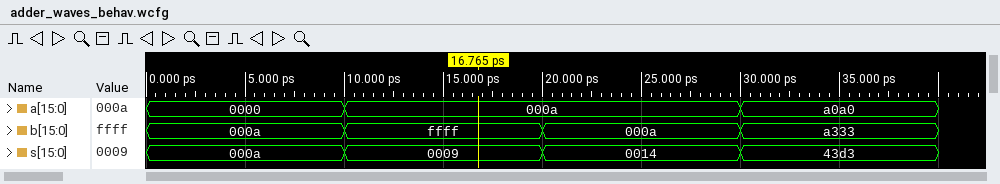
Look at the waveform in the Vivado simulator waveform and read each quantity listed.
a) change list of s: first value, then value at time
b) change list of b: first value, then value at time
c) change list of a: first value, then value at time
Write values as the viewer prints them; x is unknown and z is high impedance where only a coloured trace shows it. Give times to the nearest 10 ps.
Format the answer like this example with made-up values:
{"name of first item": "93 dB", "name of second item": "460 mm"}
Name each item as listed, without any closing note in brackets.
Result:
{"change list of s: first value, then value at time": "000a, 0009 at 10 ps, 0014 at 20 ps, 43d3 at 30 ps", "change list of b: first value, then value at time": "000a, ffff at 10 ps, 000a at 20 ps, a333 at 30 ps", "change list of a: first value, then value at time": "0000, 000a at 10 ps, a0a0 at 30 ps"}
